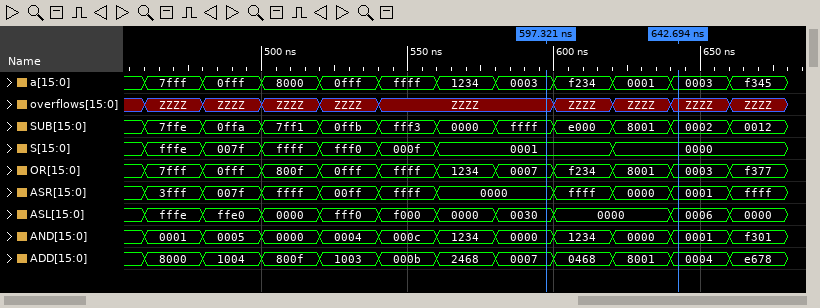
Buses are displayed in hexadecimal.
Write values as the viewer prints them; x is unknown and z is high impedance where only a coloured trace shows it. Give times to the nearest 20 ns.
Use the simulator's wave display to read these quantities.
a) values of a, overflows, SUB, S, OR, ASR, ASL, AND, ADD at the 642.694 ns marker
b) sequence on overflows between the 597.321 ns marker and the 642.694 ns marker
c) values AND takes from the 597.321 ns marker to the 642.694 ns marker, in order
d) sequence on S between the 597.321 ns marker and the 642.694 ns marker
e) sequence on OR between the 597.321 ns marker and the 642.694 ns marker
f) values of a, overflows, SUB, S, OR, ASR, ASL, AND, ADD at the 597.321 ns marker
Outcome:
a=0003, overflows=ZZZZ, SUB=0002, S=0000, OR=0003, ASR=0001, ASL=0006, AND=0001, ADD=0004
ZZZZ, ZZZZ, ZZZZ, ZZZZ
0000, 1234, 0000, 0001
0001, 0000
0007, f234, 8001, 0003
a=0003, overflows=ZZZZ, SUB=ffff, S=0001, OR=0007, ASR=0000, ASL=0030, AND=0000, ADD=0007
